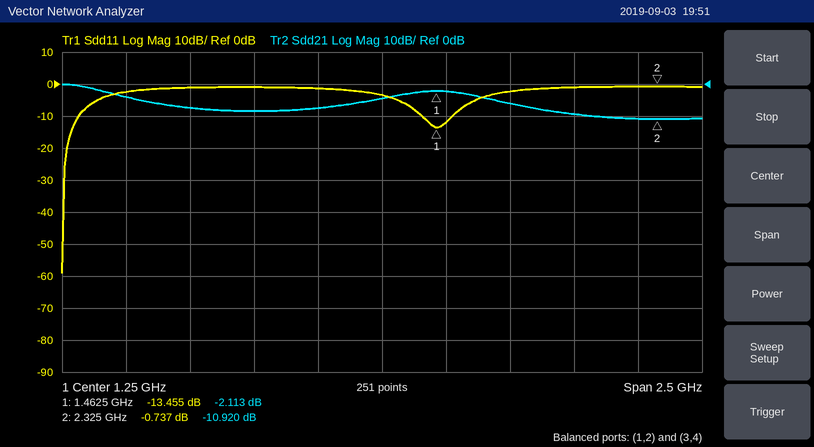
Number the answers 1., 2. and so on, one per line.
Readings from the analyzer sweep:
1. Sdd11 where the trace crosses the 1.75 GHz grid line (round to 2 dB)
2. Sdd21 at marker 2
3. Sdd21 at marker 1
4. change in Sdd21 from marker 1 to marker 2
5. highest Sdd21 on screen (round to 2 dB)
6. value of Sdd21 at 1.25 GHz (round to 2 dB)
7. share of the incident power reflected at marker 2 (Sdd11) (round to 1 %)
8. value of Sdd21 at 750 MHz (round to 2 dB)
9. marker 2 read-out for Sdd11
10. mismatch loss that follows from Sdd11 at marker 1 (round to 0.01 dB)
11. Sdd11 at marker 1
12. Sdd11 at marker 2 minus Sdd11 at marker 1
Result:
1. -2 dB
2. -10.920 dB
3. -2.113 dB
4. -8.807 dB
5. 0 dB
6. -4 dB
7. 84 %
8. -8 dB
9. -0.737 dB
10. 0.20 dB
11. -13.455 dB
12. 12.718 dB
